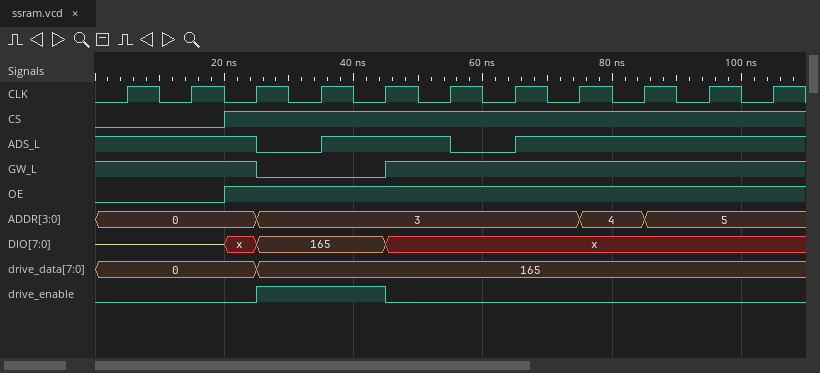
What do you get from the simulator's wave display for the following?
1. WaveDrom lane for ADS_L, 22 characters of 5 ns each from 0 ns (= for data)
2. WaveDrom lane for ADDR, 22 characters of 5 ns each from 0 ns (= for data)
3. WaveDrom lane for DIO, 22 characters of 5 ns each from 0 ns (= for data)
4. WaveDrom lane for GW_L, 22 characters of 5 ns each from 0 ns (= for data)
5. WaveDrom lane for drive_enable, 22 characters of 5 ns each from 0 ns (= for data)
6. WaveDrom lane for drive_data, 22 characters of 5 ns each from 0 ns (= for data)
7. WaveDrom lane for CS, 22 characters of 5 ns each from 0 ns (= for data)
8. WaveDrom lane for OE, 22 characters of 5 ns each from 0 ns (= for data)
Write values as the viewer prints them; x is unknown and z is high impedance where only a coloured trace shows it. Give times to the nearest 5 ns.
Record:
{name: 'ADS_L', wave: '1....0.1...0.1........'}
{name: 'ADDR', wave: '=....=.........=.=....', data: '0 3 4 5'}
{name: 'DIO', wave: 'z...x=...x............', data: '165'}
{name: 'GW_L', wave: '1....0...1............'}
{name: 'drive_enable', wave: '0....1...0............'}
{name: 'drive_data', wave: '=....=................', data: '0 165'}
{name: 'CS', wave: '0...1.................'}
{name: 'OE', wave: '0...1.................'}
